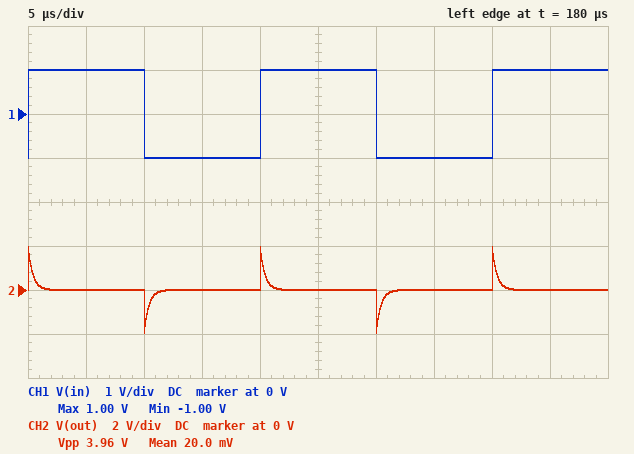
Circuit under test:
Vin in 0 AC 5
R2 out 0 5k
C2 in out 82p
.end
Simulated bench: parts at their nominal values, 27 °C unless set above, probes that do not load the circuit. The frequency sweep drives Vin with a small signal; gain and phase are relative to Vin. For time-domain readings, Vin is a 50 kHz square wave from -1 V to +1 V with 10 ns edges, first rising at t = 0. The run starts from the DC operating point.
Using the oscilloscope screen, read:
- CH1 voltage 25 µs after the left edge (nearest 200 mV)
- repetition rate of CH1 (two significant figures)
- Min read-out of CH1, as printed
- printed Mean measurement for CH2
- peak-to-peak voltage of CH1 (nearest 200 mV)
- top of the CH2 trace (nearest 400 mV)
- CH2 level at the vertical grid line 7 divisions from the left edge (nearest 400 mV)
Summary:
1.0 V
50 kHz
-1.00 V
20.0 mV
2.0 V
2.0 V
0 V
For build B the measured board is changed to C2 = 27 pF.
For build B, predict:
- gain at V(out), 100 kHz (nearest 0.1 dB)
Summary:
-21.5 dB
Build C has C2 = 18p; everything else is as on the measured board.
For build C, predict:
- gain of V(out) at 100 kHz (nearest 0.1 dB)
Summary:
-25.0 dB
